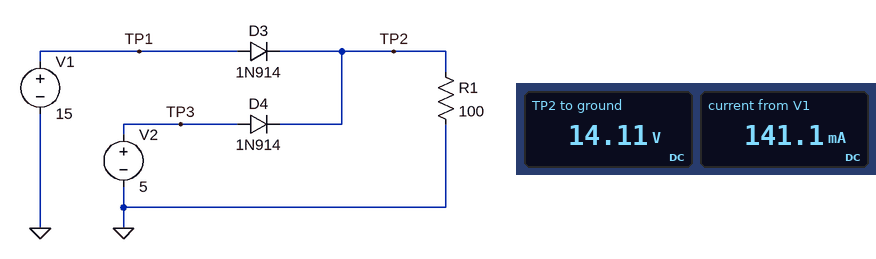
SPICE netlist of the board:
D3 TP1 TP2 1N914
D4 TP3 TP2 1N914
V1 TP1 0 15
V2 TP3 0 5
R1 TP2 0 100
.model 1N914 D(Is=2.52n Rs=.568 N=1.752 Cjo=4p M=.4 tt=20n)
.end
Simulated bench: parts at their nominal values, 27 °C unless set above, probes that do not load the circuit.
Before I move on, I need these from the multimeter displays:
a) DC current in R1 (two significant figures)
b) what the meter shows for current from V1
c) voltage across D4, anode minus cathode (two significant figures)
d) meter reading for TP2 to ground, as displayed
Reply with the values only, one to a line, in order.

140 mA
141.1 mA
-9.1 V
14.11 V
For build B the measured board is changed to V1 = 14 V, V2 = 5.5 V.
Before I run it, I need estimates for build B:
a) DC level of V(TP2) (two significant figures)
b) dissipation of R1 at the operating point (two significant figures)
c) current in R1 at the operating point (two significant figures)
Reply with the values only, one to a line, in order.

13 V
1.7 W
130 mA
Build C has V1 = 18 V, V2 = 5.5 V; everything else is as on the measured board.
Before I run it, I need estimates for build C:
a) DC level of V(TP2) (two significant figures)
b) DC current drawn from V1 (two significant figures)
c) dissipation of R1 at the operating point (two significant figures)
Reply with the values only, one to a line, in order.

17 V
170 mA
2.9 W
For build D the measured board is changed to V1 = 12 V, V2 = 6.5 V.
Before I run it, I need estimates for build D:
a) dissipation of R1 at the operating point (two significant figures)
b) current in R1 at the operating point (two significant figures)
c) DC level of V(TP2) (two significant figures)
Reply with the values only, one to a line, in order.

1.2 W
110 mA
11 V
